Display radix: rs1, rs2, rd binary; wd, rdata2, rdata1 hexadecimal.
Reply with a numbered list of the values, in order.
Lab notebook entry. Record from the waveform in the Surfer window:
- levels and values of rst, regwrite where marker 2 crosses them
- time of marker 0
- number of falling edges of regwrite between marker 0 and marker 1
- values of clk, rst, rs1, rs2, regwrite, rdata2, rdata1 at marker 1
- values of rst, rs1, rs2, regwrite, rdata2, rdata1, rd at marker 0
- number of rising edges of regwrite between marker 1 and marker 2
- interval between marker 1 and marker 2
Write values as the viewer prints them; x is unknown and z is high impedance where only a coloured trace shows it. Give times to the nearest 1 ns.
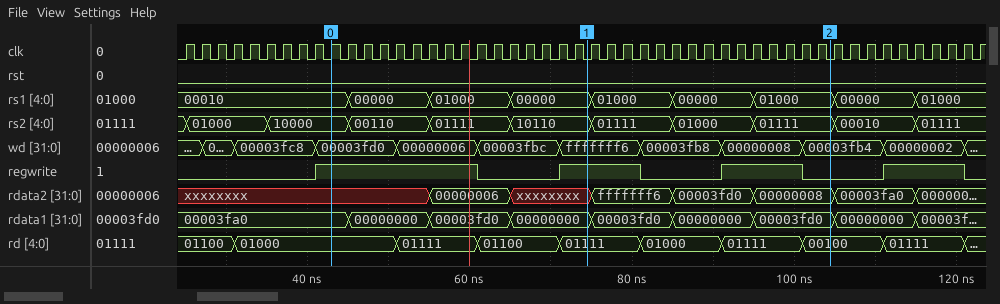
1. rst=0, regwrite=0
2. 43 ns
3. 1
4. clk=0, rst=0, rs1=00000, rs2=10110, regwrite=1, rdata2=xxxxxxxx, rdata1=00000000
5. rst=0, rs1=00010, rs2=10000, regwrite=1, rdata2=xxxxxxxx, rdata1=00003fa0, rd=01000
6. 1
7. 30 ns
